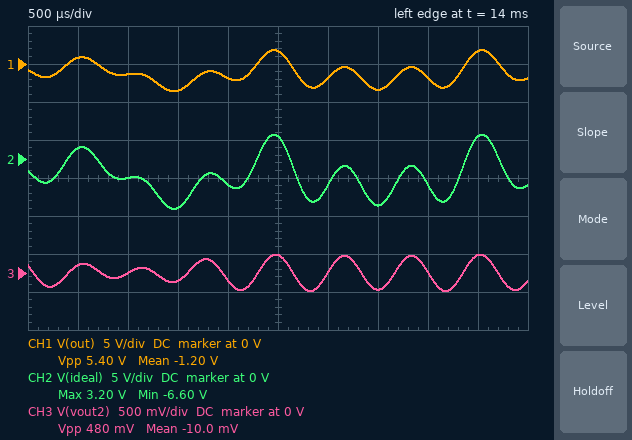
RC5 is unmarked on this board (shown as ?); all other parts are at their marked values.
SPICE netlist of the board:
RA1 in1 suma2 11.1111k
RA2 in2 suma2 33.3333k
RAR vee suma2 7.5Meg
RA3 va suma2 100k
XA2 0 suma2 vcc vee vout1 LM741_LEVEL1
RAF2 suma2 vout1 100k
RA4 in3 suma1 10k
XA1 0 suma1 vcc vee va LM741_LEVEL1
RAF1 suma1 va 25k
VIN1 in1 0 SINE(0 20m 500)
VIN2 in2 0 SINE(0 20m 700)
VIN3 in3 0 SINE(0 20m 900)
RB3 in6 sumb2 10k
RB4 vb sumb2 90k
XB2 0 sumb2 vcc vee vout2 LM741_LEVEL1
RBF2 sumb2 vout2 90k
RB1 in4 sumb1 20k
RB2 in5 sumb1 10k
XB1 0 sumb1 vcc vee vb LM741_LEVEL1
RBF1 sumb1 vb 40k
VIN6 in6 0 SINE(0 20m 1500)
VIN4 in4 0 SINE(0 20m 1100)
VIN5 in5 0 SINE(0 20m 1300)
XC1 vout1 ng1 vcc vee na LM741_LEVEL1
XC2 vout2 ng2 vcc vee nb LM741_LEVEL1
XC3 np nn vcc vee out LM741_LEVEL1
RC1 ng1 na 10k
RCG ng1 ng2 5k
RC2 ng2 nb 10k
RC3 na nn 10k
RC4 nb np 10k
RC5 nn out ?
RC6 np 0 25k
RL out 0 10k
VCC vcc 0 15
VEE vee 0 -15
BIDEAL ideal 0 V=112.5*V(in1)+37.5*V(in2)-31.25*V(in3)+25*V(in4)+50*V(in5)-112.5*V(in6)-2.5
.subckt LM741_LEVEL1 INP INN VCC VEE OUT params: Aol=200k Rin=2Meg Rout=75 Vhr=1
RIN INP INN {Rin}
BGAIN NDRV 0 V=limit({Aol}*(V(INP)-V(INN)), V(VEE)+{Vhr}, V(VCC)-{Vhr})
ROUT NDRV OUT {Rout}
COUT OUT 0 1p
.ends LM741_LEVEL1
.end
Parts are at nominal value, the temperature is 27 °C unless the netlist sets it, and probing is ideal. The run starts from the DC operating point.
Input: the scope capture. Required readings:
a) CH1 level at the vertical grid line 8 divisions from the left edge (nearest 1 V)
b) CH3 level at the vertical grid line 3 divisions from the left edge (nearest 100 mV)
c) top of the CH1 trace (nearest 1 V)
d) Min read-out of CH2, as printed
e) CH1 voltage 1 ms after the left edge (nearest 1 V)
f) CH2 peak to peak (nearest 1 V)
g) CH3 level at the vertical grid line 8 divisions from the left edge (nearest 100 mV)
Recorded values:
-2 V
-100 mV
2 V
-6.60 V
-1 V
10 V
0 V
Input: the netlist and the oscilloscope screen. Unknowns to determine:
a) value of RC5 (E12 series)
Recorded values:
12 kΩ
